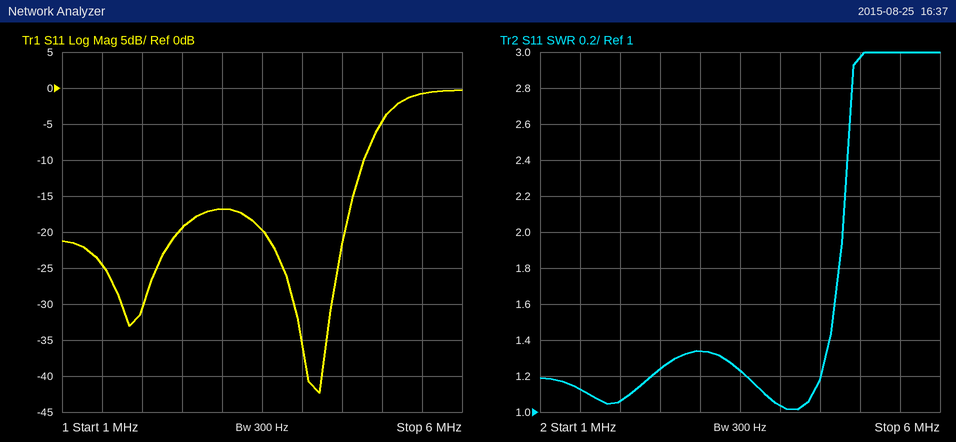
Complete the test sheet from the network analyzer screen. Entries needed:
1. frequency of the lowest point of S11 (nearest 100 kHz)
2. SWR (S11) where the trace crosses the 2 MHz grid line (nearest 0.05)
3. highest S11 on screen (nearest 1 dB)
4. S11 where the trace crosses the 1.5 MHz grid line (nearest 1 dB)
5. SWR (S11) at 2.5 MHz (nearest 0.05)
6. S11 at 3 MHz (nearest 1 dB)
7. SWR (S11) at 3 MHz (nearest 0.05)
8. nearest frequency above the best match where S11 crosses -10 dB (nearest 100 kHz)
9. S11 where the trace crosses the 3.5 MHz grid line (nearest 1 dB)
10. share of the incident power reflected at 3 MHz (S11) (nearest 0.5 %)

4.2 MHz
1.05
0 dB
-25 dB
1.25
-17 dB
1.35
4.8 MHz
-20 dB
2.0 %
